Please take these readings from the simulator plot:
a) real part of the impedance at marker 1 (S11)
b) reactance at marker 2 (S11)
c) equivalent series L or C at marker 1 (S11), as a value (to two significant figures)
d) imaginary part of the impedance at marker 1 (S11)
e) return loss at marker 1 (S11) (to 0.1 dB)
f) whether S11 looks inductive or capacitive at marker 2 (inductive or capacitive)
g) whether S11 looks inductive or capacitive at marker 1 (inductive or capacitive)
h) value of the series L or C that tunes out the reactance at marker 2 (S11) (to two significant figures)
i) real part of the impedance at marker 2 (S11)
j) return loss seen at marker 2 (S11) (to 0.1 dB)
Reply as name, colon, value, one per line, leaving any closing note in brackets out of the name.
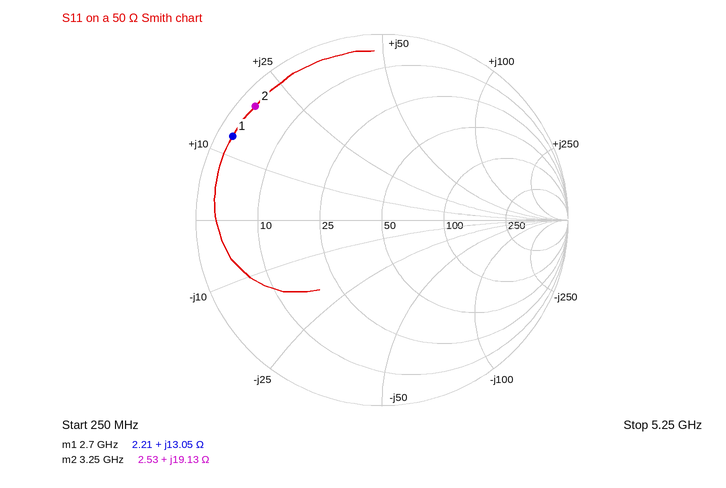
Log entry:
real part of the impedance at marker 1: 2.21 Ω
reactance at marker 2: +19.13 Ω
equivalent series L or C at marker 1 (S11), as a value: 770 pH
imaginary part of the impedance at marker 1: +13.05 Ω
return loss at marker 1 (S11): 0.7 dB
whether S11 looks inductive or capacitive at marker 2: inductive
whether S11 looks inductive or capacitive at marker 1: inductive
value of the series L or C that tunes out the reactance at marker 2 (S11): 2.6 pF
real part of the impedance at marker 2: 2.53 Ω
return loss seen at marker 2 (S11): 0.8 dB
